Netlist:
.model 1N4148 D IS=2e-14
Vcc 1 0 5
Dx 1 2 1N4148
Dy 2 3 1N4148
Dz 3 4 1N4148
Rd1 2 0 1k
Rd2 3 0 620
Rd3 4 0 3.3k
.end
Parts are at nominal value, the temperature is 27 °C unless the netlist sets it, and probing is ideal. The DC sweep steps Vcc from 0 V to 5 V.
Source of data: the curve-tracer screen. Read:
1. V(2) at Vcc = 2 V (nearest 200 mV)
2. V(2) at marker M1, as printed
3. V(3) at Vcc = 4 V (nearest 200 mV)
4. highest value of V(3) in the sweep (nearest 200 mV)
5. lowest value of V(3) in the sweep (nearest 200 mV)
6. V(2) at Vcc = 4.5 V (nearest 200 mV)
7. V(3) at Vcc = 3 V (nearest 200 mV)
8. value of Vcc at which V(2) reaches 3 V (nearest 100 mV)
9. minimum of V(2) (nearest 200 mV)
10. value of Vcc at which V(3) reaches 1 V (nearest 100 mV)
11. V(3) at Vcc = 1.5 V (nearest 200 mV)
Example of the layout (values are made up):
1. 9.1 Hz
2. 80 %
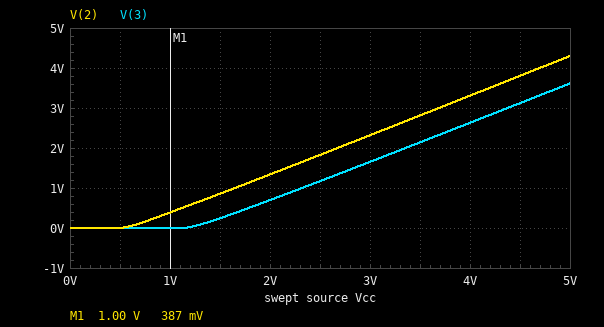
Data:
1. 1.4 V
2. 387 mV
3. 2.6 V
4. 3.6 V
5. 0 V
6. 3.8 V
7. 1.6 V
8. 3.7 V
9. 0 V
10. 2.3 V
11. 200 mV
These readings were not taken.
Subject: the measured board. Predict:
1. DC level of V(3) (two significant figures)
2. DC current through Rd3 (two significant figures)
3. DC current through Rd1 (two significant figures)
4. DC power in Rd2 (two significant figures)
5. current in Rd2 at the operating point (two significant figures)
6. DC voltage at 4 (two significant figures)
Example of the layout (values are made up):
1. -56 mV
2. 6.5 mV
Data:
1. 3.6 V
2. 900 µA
3. 4.3 mA
4. 21 mW
5. 5.8 mA
6. 3.0 V
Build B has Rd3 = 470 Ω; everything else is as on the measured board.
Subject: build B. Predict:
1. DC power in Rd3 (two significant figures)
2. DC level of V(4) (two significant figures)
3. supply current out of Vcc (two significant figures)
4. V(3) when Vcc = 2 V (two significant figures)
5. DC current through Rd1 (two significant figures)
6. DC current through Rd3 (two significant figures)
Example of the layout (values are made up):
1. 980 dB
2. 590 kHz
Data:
1. 18 mW
2. 2.9 V
3. 16 mA
4. 690 mV
5. 4.3 mA
6. 6.2 mA
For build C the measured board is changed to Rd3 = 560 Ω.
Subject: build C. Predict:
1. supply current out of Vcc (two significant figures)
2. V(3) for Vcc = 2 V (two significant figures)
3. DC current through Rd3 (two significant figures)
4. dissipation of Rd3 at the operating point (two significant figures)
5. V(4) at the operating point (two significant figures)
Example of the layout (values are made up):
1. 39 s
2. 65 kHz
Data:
1. 15 mA
2. 690 mV
3. 5.2 mA
4. 15 mW
5. 2.9 V
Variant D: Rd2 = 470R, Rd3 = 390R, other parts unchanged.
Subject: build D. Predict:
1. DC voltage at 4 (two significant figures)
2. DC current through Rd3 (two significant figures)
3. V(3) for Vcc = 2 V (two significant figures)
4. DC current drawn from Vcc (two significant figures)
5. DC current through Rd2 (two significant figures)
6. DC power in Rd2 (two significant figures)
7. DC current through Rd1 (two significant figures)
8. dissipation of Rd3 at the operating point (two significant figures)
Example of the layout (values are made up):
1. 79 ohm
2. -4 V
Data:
1. 2.9 V
2. 7.4 mA
3. 680 mV
4. 19 mA
5. 7.6 mA
6. 27 mW
7. 4.3 mA
8. 21 mW
